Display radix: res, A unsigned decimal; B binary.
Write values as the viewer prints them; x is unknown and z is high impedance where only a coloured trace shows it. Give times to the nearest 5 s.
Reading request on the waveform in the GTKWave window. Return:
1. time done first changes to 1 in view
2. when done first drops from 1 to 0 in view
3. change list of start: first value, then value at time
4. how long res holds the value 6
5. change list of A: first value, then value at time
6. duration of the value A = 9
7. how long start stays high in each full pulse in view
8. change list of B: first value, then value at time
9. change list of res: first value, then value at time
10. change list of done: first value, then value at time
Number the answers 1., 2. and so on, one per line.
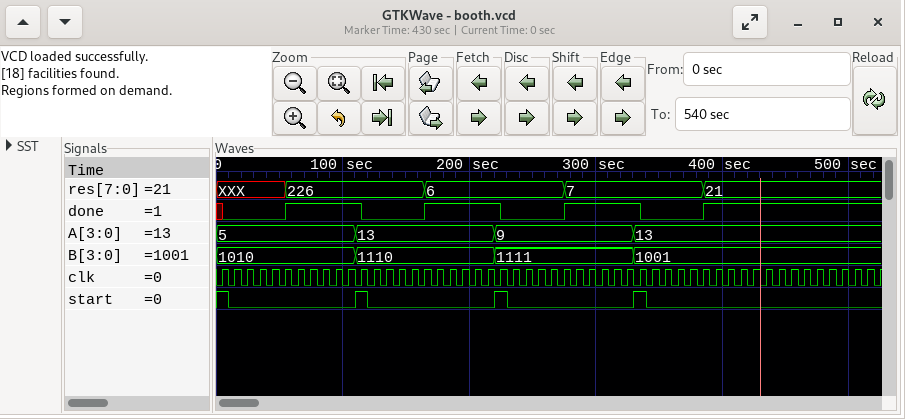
1. 55 s
2. 115 s
3. 1, 0 at 10 s, 1 at 110 s, 0 at 120 s, 1 at 220 s, 0 at 230 s, 1 at 330 s, 0 at 340 s
4. 110 s
5. 5, 13 at 110 s, 9 at 220 s, 13 at 330 s
6. 110 s
7. 10 s, 10 s, 10 s
8. 1010, 1110 at 110 s, 1111 at 220 s, 1001 at 330 s
9. XXX, 226 at 55 s, 6 at 165 s, 7 at 275 s, 21 at 385 s
10. x, 0 at 5 s, 1 at 55 s, 0 at 115 s, 1 at 165 s, 0 at 225 s, 1 at 275 s, 0 at 335 s, 1 at 385 s
